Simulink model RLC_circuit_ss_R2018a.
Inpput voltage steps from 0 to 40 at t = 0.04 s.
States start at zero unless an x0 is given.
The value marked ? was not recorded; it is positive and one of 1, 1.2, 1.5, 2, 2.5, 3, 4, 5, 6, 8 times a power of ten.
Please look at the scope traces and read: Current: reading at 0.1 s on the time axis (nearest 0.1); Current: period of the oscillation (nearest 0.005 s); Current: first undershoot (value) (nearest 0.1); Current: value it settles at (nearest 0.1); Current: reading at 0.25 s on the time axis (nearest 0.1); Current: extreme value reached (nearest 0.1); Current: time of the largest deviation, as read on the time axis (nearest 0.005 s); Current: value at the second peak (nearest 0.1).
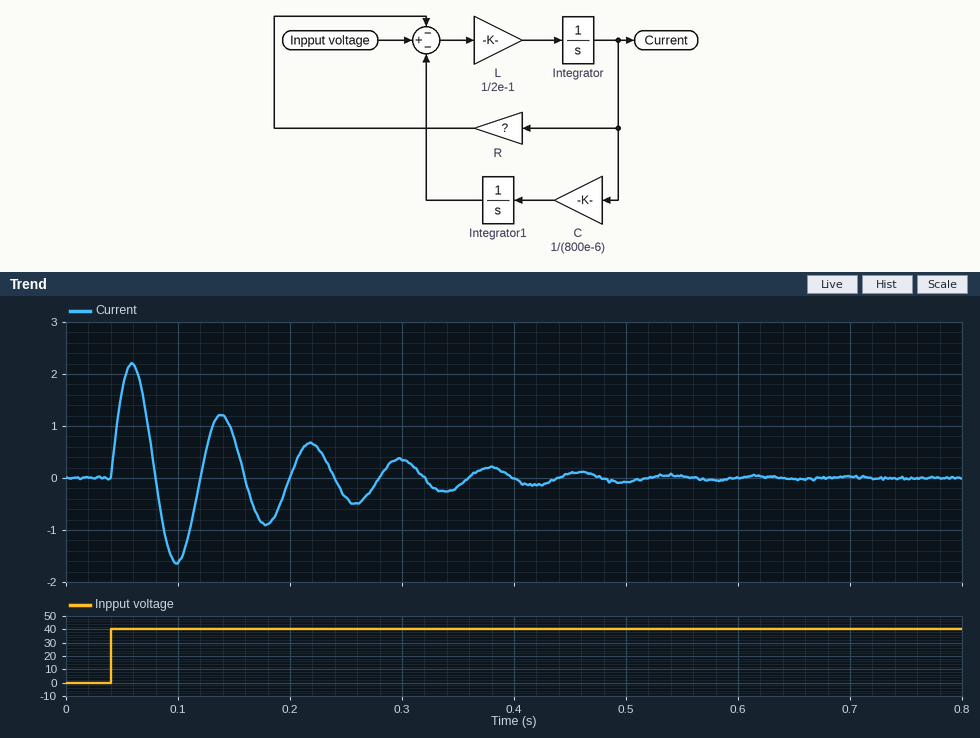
-1.6
0.080 s
-1.6
0.0
-0.4
2.2
0.060 s
1.2
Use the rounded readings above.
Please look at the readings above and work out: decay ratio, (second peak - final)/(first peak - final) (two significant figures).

0.55
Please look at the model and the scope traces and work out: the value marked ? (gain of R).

3
